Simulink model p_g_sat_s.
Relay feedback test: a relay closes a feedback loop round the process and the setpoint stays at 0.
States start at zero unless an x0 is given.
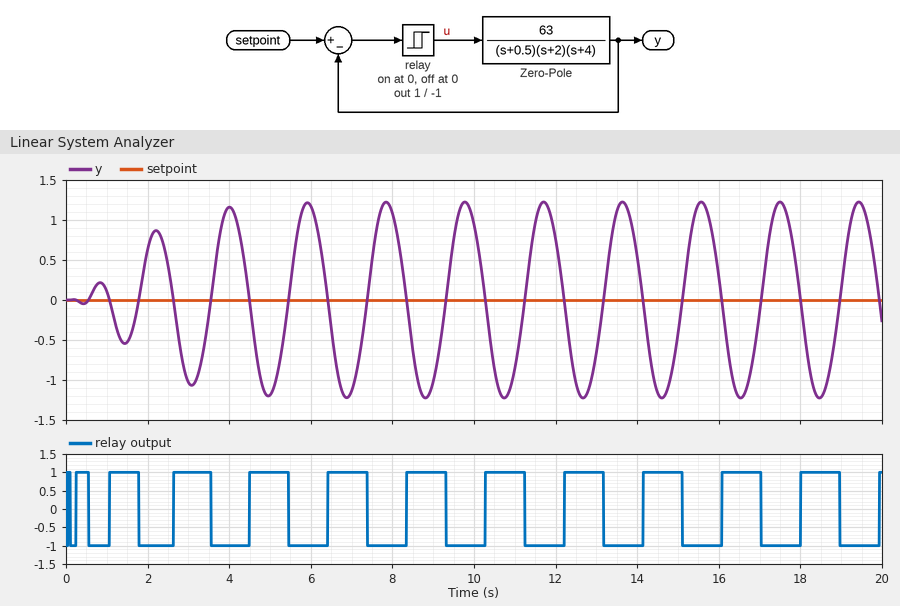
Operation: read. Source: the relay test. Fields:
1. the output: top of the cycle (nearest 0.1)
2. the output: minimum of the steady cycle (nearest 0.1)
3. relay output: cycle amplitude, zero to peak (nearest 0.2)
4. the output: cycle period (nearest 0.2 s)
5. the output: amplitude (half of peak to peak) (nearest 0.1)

1.2
-1.2
1.0
2.0 s
1.2
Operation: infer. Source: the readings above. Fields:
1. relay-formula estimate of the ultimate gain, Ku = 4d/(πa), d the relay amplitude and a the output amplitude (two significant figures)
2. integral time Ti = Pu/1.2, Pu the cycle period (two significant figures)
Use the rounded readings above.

1.1
1.7 s
